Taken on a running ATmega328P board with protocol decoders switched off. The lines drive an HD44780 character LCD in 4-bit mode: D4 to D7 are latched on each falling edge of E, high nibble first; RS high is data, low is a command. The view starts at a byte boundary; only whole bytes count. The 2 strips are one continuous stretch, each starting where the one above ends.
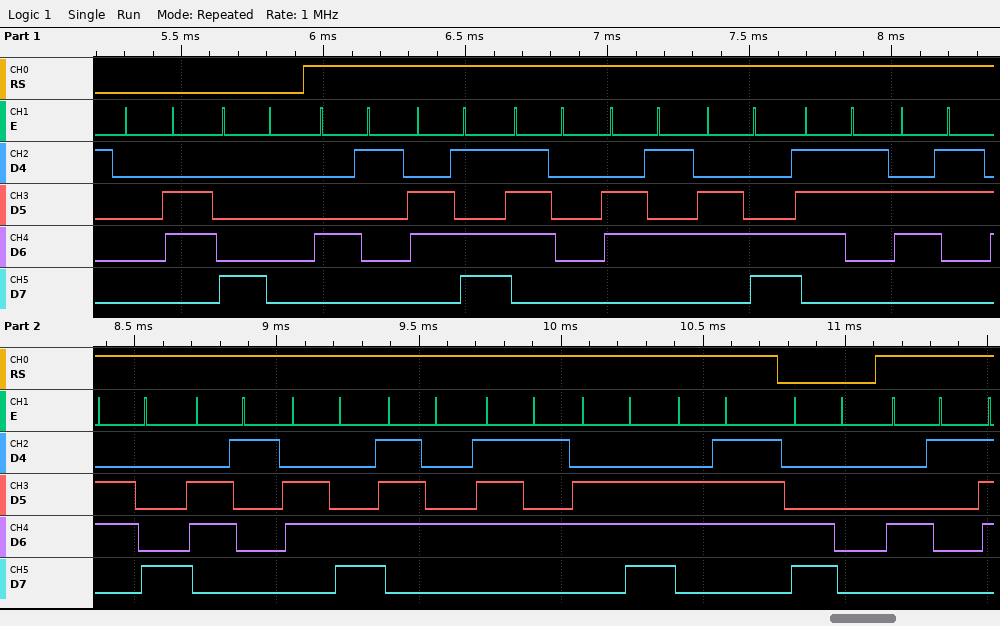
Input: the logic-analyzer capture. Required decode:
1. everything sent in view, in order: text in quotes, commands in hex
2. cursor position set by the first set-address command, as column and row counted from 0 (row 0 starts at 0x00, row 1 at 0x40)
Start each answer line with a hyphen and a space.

- 0x06 0x80 "Ampelschaltung" 0xC0 "A"
- column 0, row 0
